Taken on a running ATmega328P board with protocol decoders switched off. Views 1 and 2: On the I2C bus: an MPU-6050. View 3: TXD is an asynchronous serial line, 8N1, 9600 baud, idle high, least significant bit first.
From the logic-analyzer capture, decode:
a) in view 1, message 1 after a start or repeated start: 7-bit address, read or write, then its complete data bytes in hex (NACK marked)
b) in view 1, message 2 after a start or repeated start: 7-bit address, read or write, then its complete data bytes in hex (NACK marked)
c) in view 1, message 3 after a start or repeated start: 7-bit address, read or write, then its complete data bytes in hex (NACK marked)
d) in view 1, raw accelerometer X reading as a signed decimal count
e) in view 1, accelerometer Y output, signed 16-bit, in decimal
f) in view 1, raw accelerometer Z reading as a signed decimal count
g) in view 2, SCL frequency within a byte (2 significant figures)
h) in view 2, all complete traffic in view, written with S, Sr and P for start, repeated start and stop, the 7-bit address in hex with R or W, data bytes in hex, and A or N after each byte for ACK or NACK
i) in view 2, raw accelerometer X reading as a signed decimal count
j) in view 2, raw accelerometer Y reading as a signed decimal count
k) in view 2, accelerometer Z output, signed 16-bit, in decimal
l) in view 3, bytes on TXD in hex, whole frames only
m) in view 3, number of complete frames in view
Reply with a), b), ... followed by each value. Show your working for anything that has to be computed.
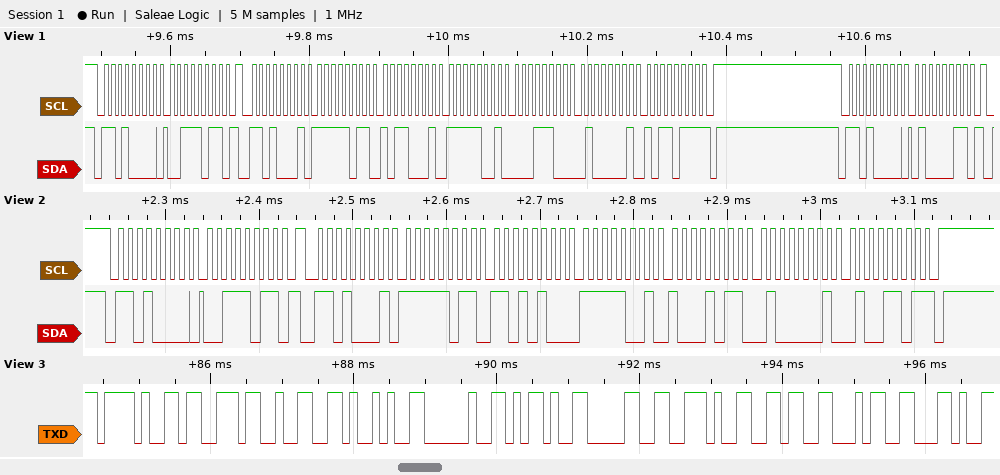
a) 0x68 write: 3B
b) 0x68 read: FB B1 F9 1C 41 B7 NACK
c) 0x68 write: 43
d) 0xFBB1 = -1103
e) 0xF91C = -1764
f) 0x41B7 = 16823
g) 100 kHz
h) S 68W A 3B A Sr 68R A FB A D4 A F9 A 8B A 41 A 4D N P
i) 0xFBD4 = -1068
j) 0xF98B = -1653
k) 0x414D = 16717
l) 0x2F 0x73 0x32 0x29 0x20 0x2D 0x30 0x2E 0x36 0x34 0x2C
m) 11
